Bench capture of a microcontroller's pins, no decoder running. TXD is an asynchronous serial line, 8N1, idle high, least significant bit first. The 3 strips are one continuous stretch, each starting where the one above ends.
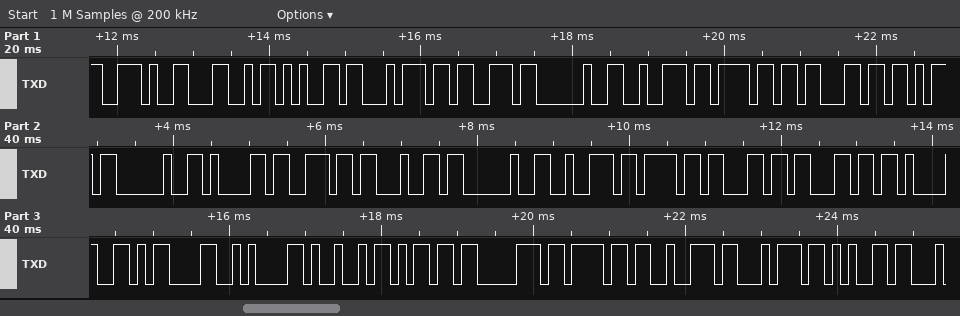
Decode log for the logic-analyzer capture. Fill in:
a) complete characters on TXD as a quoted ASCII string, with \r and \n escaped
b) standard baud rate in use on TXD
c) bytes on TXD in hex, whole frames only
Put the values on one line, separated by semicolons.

".Lets rock and roll!\r\nImporte"; 9600 baud; 2E 4C 65 74 73 20 72 6F 63 6B 20 61 6E 64 20 72 6F 6C 6C 21 0D 0A 49 6D 70 6F 72 74 65
